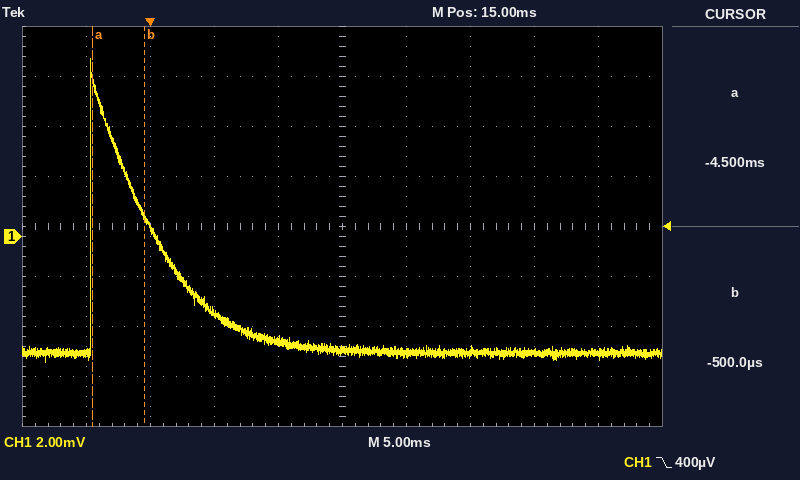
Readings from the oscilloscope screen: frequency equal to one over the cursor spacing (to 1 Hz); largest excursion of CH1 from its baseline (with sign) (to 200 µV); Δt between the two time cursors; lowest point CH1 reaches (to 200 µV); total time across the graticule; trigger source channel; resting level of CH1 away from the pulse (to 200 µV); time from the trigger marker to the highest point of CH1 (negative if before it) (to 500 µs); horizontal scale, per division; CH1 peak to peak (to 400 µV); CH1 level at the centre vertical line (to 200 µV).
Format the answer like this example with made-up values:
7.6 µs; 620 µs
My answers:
250 Hz; +11.8 mV; 4.0 ms; -5.0 mV; 50 ms; CH1; -4.6 mV; -4.5 ms; 5 ms; 12.0 mV; -4.6 mV
